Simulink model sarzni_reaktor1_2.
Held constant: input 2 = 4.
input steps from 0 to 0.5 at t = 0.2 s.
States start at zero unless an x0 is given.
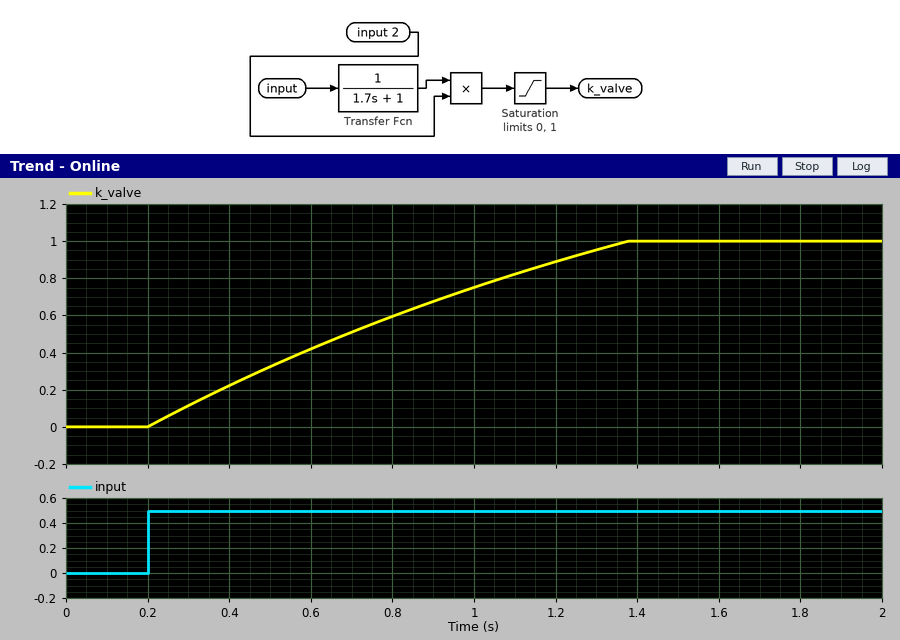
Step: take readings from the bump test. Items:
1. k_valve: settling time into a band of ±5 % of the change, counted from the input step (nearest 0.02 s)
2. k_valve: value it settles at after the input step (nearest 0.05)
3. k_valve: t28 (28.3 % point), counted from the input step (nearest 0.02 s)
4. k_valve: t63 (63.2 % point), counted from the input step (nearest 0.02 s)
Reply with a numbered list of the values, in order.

1. 1.10 s
2. 1.00
3. 0.26 s
4. 0.64 s
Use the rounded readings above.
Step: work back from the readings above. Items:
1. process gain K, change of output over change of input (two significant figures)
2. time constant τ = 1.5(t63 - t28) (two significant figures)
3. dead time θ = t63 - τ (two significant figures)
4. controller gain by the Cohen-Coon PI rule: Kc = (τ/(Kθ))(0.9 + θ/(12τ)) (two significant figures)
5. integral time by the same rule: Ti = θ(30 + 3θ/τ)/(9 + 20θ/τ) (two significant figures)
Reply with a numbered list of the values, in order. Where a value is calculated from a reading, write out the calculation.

1. (1 - 0) / 0.5 = 2.0
2. 1.5 × (0.64 - 0.26) = 0.57 s
3. 0.64 - 0.57 = 0.070 s
4. 0.57 / (2 × 0.07) × (0.9 + 0.07 / (12 × 0.57)) = 3.7
5. 0.07 × (30 + 3 × 0.07 / 0.57) / (9 + 20 × 0.07 / 0.57) = 0.19 s
